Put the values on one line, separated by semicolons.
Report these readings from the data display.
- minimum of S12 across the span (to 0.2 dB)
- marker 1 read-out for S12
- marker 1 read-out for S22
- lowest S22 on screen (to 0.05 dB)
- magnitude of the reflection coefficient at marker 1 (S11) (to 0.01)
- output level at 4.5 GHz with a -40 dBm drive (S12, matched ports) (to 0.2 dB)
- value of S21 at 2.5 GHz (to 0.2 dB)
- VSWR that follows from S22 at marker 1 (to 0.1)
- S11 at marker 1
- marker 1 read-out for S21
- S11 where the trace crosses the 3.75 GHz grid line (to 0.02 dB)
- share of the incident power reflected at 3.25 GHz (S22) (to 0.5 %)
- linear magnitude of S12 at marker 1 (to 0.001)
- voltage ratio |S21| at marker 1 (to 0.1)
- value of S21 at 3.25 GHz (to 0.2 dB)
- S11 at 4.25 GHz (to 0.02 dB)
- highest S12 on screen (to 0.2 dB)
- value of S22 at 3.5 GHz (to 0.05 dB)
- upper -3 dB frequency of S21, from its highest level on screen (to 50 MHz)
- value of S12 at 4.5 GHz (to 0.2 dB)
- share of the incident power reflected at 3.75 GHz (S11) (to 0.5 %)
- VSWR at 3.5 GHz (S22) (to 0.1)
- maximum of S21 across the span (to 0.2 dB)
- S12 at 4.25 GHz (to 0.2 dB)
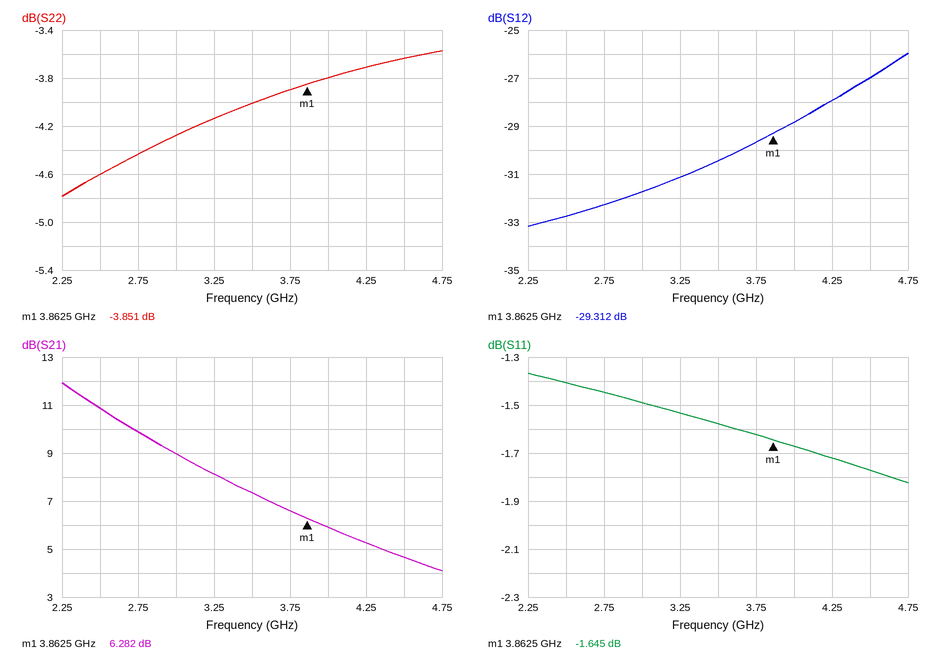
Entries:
-33.2 dB; -29.312 dB; -3.851 dB; -4.80 dB; 0.83; -67.0 dBm; 10.8 dB; 4.6; -1.645 dB; 6.282 dB; -1.62 dB; 38.5 %; 0.034; 2.1; 8.2 dB; -1.72 dB; -26.0 dB; -4.00 dB; 3.00 GHz; -27.0 dB; 69.0 %; 4.4; 12.0 dB; -28.0 dB
